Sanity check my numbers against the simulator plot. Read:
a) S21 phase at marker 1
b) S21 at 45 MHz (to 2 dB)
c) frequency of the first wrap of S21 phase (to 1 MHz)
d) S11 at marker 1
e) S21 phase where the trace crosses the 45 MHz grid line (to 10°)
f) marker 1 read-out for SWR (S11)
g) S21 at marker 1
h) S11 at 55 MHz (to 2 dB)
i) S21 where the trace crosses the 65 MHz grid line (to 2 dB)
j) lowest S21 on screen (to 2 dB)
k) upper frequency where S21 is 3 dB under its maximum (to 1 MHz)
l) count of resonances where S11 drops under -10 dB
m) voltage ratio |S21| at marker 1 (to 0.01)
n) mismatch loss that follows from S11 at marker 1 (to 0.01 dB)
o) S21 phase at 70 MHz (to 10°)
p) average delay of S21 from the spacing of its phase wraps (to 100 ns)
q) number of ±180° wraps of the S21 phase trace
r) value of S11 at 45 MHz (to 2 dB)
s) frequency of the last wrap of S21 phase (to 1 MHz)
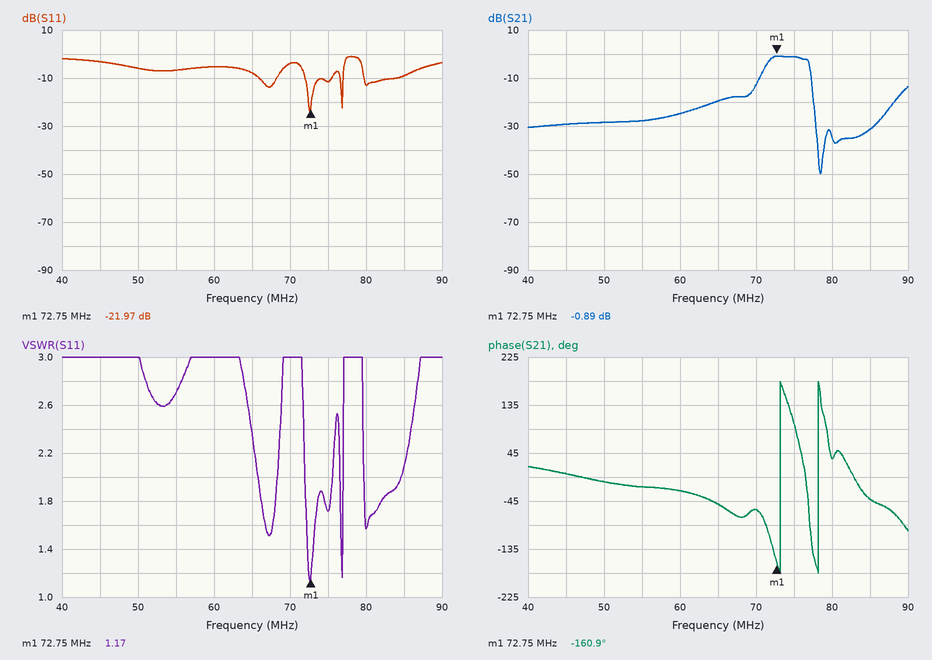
-160.9°
-30 dB
73 MHz
-21.97 dB
10°
1.17
-0.89 dB
-6 dB
-20 dB
-50 dB
77 MHz
4
0.90
0.03 dB
-60°
200 ns
2
-4 dB
78 MHz
